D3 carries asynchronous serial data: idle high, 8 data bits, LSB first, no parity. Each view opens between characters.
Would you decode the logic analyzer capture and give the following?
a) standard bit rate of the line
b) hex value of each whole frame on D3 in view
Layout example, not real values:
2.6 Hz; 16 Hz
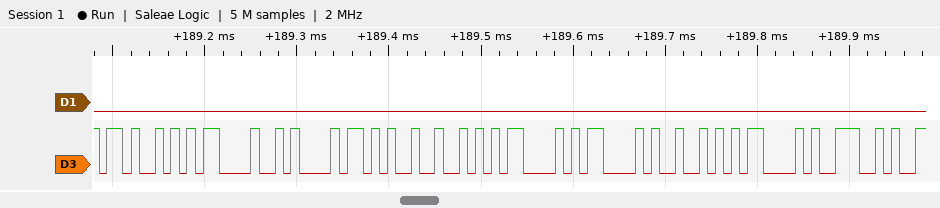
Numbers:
115200 baud; 4B, 0D, 0A, 2B, 52, 43, 43, 52, 43, 4E
